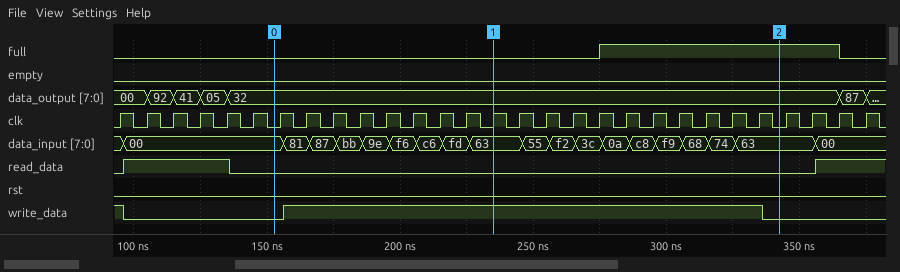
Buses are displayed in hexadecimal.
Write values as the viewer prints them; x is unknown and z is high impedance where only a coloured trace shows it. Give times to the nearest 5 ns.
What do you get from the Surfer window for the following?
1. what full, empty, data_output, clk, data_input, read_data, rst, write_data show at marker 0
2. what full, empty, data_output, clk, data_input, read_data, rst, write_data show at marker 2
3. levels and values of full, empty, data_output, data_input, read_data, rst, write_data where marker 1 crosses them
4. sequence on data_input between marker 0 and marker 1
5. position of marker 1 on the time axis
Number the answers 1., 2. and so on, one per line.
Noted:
1. full=0, empty=0, data_output=32, clk=0, data_input=00, read_data=0, rst=0, write_data=0
2. full=1, empty=0, data_output=32, clk=0, data_input=63, read_data=0, rst=0, write_data=0
3. full=0, empty=0, data_output=32, data_input=63, read_data=0, rst=0, write_data=1
4. 00, 81, 87, bb, 9e, f6, c6, fd, 63
5. 235 ns
